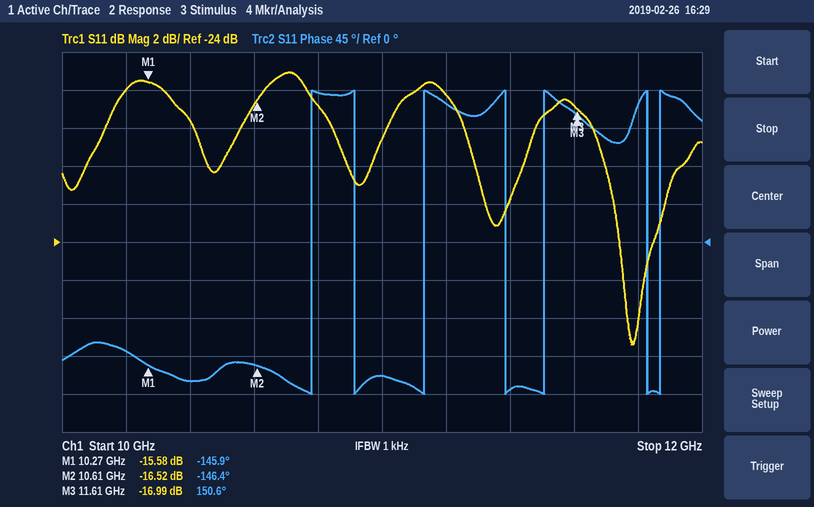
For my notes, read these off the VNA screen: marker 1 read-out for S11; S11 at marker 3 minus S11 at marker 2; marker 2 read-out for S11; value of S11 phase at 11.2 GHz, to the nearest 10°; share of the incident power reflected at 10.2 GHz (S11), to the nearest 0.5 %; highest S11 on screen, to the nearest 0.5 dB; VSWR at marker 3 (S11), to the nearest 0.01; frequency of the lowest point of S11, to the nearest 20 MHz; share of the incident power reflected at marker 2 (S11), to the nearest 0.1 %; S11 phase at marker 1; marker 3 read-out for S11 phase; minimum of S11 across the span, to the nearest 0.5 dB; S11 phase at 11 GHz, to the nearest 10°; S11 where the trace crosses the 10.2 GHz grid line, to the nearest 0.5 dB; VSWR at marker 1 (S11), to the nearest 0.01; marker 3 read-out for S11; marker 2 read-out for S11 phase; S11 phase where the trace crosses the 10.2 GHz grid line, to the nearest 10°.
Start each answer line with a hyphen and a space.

- -15.58 dB
- -0.47 dB
- -16.52 dB
- 160°
- 2.5 %
- -15.0 dB
- 1.33
- 11.78 GHz
- 2.2 %
- -145.9°
- 150.6°
- -29.5 dB
- -160°
- -16.0 dB
- 1.40
- -16.99 dB
- -146.4°
- -130°
